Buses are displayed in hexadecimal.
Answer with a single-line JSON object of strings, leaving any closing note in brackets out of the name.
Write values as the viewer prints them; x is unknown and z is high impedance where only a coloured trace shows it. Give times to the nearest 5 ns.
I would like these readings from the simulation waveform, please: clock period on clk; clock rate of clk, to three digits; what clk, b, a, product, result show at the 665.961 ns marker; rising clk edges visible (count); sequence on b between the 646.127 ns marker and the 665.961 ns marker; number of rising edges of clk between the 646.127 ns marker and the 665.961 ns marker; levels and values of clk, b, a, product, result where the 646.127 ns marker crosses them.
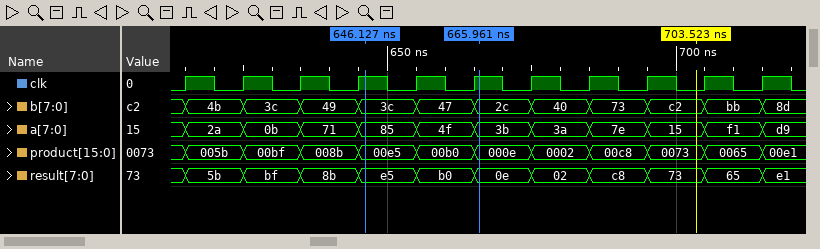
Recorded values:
{"clock period on clk": "10 ns", "clock rate of clk, to three digits": "100 MHz", "what clk, b, a, product, result show at the 665.961 ns marker": "clk=1, b=2c, a=3b, product=000e, result=0e", "rising clk edges visible": "11", "sequence on b between the 646.127 ns marker and the 665.961 ns marker": "3c, 47, 2c", "number of rising edges of clk between the 646.127 ns marker and the 665.961 ns marker": "2", "levels and values of clk, b, a, product, result where the 646.127 ns marker crosses them": "clk=1, b=3c, a=85, product=00e5, result=e5"}
